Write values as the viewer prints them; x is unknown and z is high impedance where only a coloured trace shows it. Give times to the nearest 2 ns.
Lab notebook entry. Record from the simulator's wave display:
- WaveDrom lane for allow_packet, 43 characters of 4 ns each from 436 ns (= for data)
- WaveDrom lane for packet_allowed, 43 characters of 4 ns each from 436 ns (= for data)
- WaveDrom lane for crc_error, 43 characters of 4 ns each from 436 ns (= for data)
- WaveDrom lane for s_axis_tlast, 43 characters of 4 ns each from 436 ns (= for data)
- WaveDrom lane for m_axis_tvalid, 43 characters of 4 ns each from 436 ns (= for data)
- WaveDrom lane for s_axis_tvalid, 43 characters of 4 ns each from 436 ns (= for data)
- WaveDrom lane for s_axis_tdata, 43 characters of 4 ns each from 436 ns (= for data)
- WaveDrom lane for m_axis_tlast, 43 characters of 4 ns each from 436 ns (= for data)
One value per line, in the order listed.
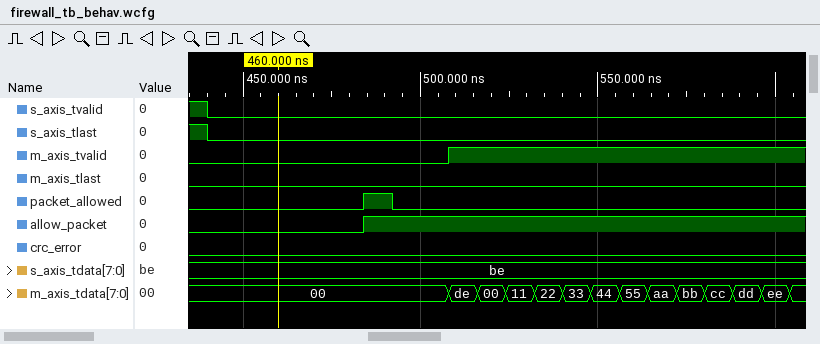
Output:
{name: 'allow_packet', wave: '0...........1..............................'}
{name: 'packet_allowed', wave: '0...........1.0............................'}
{name: 'crc_error', wave: '0..........................................'}
{name: 's_axis_tlast', wave: '10.........................................'}
{name: 'm_axis_tvalid', wave: '0.................1........................'}
{name: 's_axis_tvalid', wave: '10.........................................'}
{name: 's_axis_tdata', wave: '=..........................................', data: 'be'}
{name: 'm_axis_tlast', wave: '0..........................................'}
